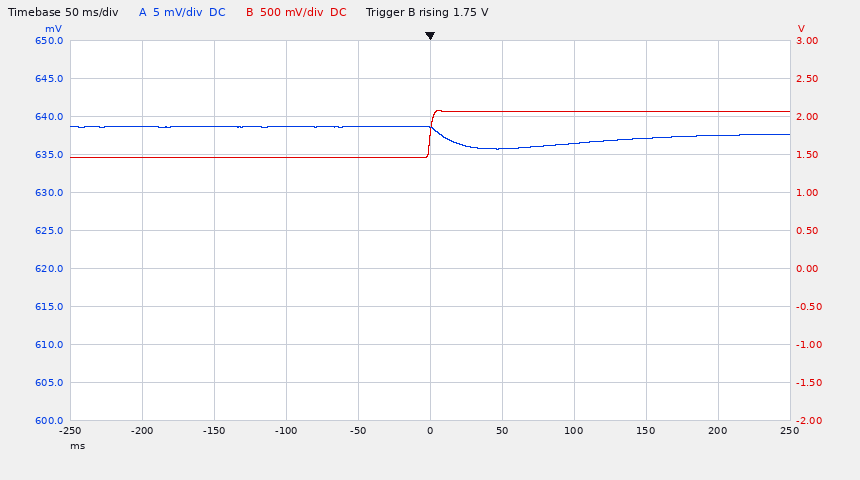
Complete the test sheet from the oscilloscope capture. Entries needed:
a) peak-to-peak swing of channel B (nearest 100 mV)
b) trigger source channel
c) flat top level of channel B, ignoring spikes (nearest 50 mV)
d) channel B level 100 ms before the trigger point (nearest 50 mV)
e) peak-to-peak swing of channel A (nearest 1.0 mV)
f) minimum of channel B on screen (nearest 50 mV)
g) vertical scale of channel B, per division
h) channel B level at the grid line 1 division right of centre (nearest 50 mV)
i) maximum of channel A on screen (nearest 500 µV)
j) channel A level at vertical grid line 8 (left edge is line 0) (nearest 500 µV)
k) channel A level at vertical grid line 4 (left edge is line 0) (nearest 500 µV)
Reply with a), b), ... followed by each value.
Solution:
a) 600 mV
b) channel B
c) 2.05 V
d) 1.45 V
e) 3.0 mV
f) 1.45 V
g) 500 mV
h) 2.05 V
i) 638.5 mV
j) 637.0 mV
k) 638.5 mV
